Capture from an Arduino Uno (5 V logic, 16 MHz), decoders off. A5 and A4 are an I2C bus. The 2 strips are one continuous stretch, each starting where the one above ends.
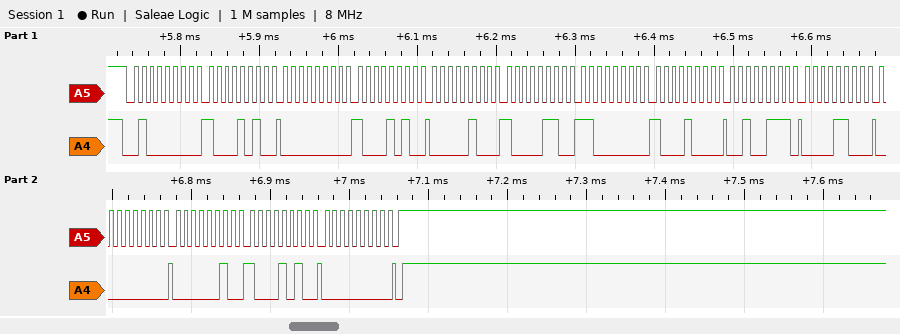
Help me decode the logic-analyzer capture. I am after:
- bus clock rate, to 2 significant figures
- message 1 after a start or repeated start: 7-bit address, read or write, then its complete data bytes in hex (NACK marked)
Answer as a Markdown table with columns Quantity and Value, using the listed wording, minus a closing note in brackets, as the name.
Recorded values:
| Quantity | Value |
|---|---|
| bus clock rate, to 2 significant figures | 100 kHz |
| message 1 after a start or repeated start: 7-bit address, read or write, then its complete data bytes in hex | 0x20 write: 8A 00 8A 04 86 C0 88 27 0C 00 02 8A 00 |
